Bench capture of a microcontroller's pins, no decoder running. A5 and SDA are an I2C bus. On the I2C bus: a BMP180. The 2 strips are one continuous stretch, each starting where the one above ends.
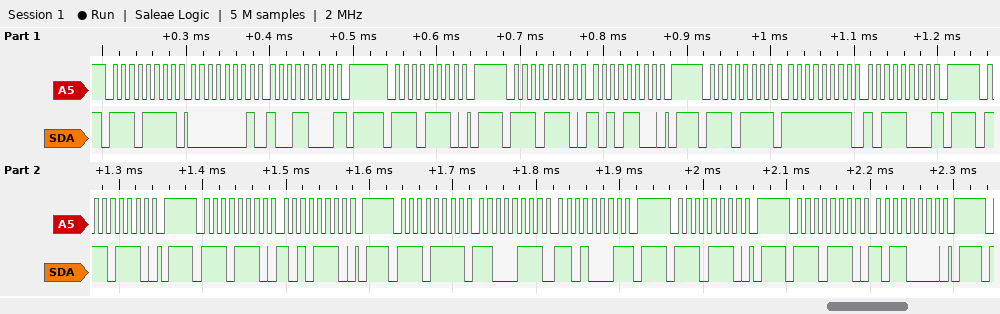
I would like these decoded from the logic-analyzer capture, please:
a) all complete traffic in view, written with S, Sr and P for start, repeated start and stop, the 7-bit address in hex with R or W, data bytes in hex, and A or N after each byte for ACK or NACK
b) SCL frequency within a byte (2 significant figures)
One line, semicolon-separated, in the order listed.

S 77R A 01 A 98 N P S 77W A P S 77W A AC A P S 77R A FF A B8 N P S 77W A P S 77W A AE A P S 77R A C7 A D1 N P S 77W A P S 77W A B0 A P; 100 kHz
